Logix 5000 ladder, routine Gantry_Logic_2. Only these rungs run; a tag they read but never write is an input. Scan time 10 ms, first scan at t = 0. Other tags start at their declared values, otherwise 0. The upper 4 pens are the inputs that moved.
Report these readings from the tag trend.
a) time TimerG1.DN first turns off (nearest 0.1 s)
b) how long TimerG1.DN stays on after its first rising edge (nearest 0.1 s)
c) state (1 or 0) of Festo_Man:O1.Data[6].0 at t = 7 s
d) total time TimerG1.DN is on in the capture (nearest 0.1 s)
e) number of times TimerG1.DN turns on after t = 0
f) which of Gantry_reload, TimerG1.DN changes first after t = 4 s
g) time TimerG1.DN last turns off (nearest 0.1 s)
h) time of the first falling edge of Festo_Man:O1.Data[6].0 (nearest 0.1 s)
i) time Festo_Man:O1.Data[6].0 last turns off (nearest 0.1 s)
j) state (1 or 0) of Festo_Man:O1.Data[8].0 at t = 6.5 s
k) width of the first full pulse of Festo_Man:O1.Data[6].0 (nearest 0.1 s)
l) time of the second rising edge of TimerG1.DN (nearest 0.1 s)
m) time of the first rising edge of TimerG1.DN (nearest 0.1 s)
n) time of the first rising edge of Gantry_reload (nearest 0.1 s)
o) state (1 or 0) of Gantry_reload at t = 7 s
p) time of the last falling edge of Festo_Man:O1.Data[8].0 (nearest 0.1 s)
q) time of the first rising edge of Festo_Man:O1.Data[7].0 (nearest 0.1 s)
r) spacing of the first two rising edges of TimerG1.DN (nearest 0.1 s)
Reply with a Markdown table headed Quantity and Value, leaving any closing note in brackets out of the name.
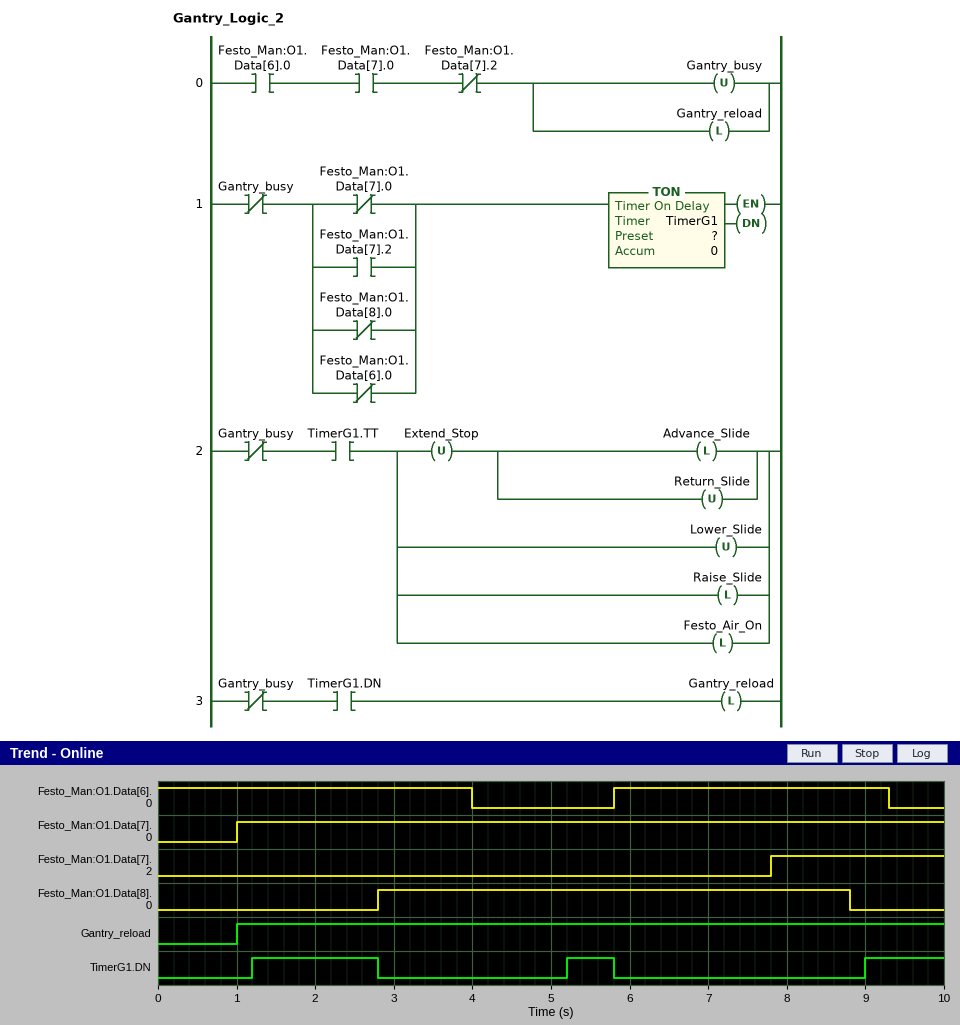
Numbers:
| Quantity | Value |
|---|---|
| time TimerG1.DN first turns off | 2.8 s |
| how long TimerG1.DN stays on after its first rising edge | 1.6 s |
| state (1 or 0) of Festo_Man:O1.Data[6].0 at t = 7 s | 1 |
| total time TimerG1.DN is on in the capture | 3.2 s |
| number of times TimerG1.DN turns on after t = 0 | 3 |
| which of Gantry_reload, TimerG1.DN changes first after t = 4 s | TimerG1.DN |
| time TimerG1.DN last turns off | 5.8 s |
| time of the first falling edge of Festo_Man:O1.Data[6].0 | 4.0 s |
| time Festo_Man:O1.Data[6].0 last turns off | 9.3 s |
| state (1 or 0) of Festo_Man:O1.Data[8].0 at t = 6.5 s | 1 |
| width of the first full pulse of Festo_Man:O1.Data[6].0 | 3.5 s |
| time of the second rising edge of TimerG1.DN | 5.2 s |
| time of the first rising edge of TimerG1.DN | 1.2 s |
| time of the first rising edge of Gantry_reload | 1.0 s |
| state (1 or 0) of Gantry_reload at t = 7 s | 1 |
| time of the last falling edge of Festo_Man:O1.Data[8].0 | 8.8 s |
| time of the first rising edge of Festo_Man:O1.Data[7].0 | 1.0 s |
| spacing of the first two rising edges of TimerG1.DN | 4.0 s |
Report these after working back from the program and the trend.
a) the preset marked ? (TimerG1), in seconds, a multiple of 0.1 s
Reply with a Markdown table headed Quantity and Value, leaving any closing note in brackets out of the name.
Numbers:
| Quantity | Value |
|---|---|
| the preset marked ? (TimerG1), in seconds, a multiple of 0.1 s | 1.2 s |
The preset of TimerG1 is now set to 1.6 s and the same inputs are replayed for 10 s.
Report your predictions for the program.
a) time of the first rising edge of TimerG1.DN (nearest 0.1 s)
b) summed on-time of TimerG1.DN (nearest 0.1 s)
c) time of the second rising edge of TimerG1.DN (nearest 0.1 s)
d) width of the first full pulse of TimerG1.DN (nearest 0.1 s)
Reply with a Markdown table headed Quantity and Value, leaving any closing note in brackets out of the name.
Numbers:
| Quantity | Value |
|---|---|
| time of the first rising edge of TimerG1.DN | 1.6 s |
| summed on-time of TimerG1.DN | 2.0 s |
| time of the second rising edge of TimerG1.DN | 5.6 s |
| width of the first full pulse of TimerG1.DN | 1.2 s |
